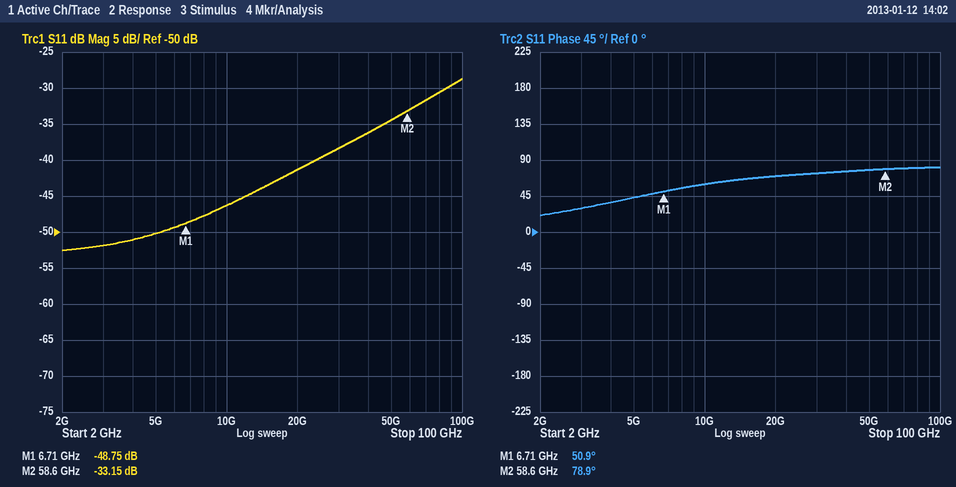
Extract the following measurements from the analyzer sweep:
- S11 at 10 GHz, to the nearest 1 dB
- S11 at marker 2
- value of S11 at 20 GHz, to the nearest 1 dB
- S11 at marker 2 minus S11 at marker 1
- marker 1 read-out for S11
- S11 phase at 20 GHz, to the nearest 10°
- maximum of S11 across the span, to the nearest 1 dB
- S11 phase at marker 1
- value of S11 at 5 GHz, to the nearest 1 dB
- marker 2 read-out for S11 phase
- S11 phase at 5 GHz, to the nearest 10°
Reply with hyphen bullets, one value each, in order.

- -46 dB
- -33.15 dB
- -41 dB
- 15.60 dB
- -48.75 dB
- 70°
- -29 dB
- 50.9°
- -50 dB
- 78.9°
- 40°
